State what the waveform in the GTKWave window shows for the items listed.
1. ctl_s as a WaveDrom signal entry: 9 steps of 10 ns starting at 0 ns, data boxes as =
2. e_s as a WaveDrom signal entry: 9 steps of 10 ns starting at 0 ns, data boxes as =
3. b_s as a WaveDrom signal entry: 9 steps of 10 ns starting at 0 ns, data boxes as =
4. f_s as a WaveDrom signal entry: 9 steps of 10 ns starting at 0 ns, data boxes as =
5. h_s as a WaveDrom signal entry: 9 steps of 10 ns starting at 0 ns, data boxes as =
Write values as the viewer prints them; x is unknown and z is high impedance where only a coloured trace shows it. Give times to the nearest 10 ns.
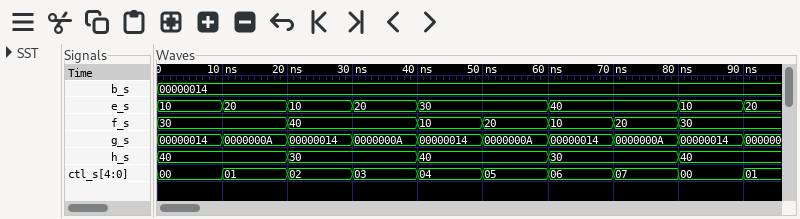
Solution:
{name: 'ctl_s', wave: '=========', data: '00 01 02 03 04 05 06 07 00'}
{name: 'e_s', wave: '=====.=.=', data: '10 20 10 20 30 40 10'}
{name: 'b_s', wave: '=........', data: '00000014'}
{name: 'f_s', wave: '=.=.=====', data: '30 40 10 20 10 20 30'}
{name: 'h_s', wave: '=.=.=.=.=', data: '40 30 40 30 40'}
